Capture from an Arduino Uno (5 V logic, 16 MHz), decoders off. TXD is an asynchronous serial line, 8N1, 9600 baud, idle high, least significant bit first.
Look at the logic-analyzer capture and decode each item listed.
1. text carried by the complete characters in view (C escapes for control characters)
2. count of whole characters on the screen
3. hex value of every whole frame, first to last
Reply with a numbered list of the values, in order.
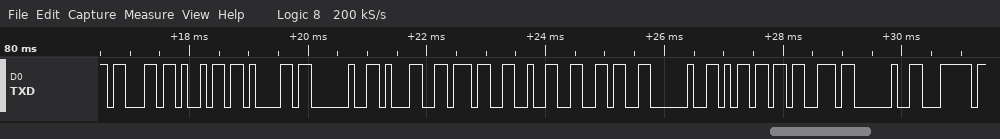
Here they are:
1. "cia 1726 ms |"
2. 13
3. 63 69 61 20 31 37 32 36 20 6D 73 20 7C
